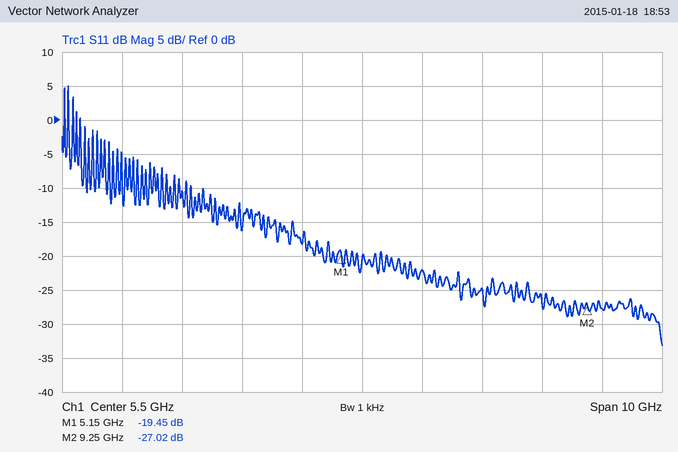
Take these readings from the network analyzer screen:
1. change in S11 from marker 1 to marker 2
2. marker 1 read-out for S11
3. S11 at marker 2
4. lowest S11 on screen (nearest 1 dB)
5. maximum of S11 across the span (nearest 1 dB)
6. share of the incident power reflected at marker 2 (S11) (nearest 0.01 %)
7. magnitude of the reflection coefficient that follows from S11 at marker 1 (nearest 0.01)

-7.57 dB
-19.45 dB
-27.02 dB
-33 dB
5 dB
0.20 %
0.11
